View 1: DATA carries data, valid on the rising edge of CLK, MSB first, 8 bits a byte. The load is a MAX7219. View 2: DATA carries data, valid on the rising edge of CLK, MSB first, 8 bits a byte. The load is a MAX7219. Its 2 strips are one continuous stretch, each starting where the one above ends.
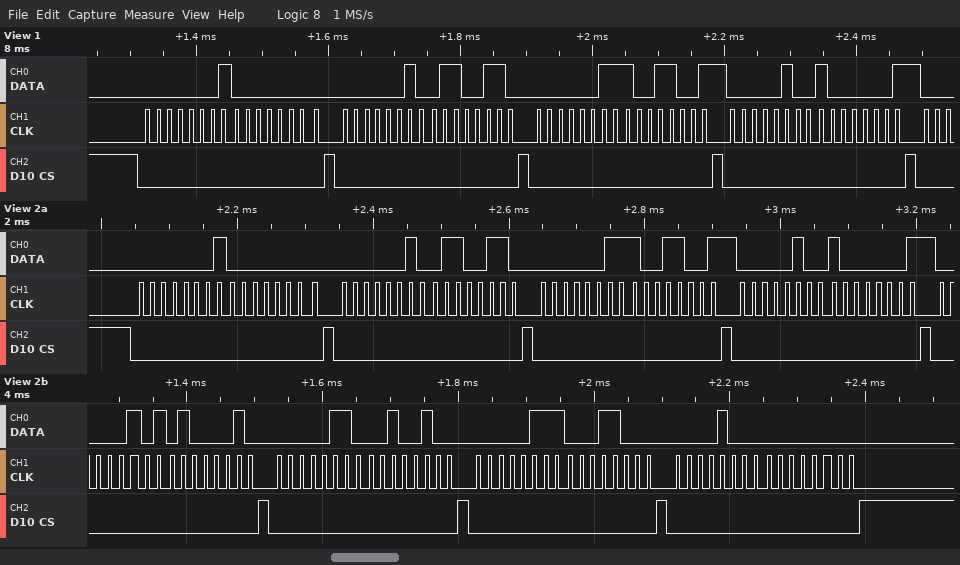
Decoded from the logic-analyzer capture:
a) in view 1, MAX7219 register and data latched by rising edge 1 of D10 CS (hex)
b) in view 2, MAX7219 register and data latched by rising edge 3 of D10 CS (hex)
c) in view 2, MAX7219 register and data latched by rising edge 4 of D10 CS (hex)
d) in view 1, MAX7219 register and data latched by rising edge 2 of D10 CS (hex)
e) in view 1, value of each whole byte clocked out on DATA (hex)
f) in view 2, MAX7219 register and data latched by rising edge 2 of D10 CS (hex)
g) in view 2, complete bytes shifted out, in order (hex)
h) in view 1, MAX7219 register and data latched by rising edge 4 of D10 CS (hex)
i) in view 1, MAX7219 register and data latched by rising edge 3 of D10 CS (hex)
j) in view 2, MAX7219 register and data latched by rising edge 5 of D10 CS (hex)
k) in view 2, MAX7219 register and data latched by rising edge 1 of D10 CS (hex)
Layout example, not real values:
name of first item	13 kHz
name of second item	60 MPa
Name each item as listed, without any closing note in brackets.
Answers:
in view 1, MAX7219 register and data latched by rising edge 1 of D10 CS	register 0x1, data 0x00
in view 2, MAX7219 register and data latched by rising edge 3 of D10 CS	register 0x3, data 0x99
in view 2, MAX7219 register and data latched by rising edge 4 of D10 CS	register 0x4, data 0x81
in view 1, MAX7219 register and data latched by rising edge 2 of D10 CS	register 0x2, data 0x66
in view 1, value of each whole byte clocked out on DATA	0x01 0x00 0x02 0x66 0x03 0x99 0x04 0x81
in view 2, MAX7219 register and data latched by rising edge 2 of D10 CS	register 0x2, data 0x66
in view 2, complete bytes shifted out, in order	01 00 02 66 03 99 04 81 05 42 06 24 07 18 08 00
in view 1, MAX7219 register and data latched by rising edge 4 of D10 CS	register 0x4, data 0x81
in view 1, MAX7219 register and data latched by rising edge 3 of D10 CS	register 0x3, data 0x99
in view 2, MAX7219 register and data latched by rising edge 5 of D10 CS	register 0x5, data 0x42
in view 2, MAX7219 register and data latched by rising edge 1 of D10 CS	register 0x1, data 0x00
